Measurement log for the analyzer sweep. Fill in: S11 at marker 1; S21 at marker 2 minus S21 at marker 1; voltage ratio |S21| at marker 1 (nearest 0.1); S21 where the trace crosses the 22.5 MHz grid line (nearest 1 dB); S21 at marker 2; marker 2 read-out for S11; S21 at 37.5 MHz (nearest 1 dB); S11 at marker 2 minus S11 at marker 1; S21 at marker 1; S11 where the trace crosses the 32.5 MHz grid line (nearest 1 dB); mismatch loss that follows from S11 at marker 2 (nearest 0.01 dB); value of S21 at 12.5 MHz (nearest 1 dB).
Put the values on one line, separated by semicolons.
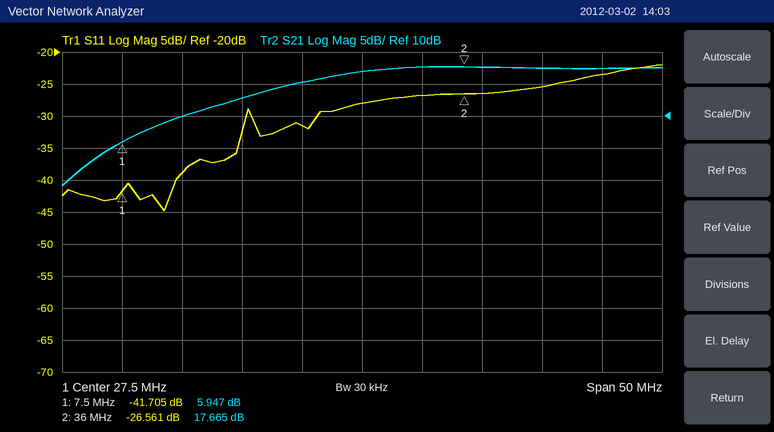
-41.705 dB; 11.718 dB; 2.0; 15 dB; 17.665 dB; -26.561 dB; 18 dB; 15.144 dB; 5.947 dB; -27 dB; 0.01 dB; 10 dB
